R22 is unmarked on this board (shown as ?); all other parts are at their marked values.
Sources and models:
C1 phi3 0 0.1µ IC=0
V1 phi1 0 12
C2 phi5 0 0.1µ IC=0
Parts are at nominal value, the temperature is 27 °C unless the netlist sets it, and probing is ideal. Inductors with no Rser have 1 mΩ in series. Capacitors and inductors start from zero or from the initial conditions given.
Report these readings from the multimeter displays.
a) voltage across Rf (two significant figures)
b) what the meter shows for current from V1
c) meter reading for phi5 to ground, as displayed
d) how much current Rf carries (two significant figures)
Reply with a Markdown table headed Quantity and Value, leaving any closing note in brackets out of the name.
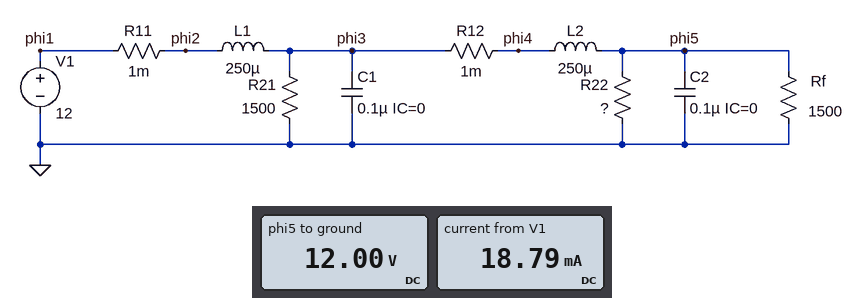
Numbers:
| Quantity | Value |
|---|---|
| voltage across Rf | 12 V |
| what the meter shows for current from V1 | 18.79 mA |
| meter reading for phi5 to ground, as displayed | 12.00 V |
| how much current Rf carries | 8.0 mA |
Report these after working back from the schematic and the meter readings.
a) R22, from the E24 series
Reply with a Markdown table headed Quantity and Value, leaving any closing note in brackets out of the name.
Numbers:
| Quantity | Value |
|---|---|
| R22, from the E24 series | 4.3 kΩ |
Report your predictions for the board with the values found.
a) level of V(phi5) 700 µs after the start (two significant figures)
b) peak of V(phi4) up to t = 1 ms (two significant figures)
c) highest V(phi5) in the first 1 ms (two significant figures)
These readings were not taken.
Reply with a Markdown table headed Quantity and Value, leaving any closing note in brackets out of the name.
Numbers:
| Quantity | Value |
|---|---|
| level of V(phi5) 700 µs after the start | 12 V |
| peak of V(phi4) up to t = 1 ms | 22 V |
| highest V(phi5) in the first 1 ms | 25 V |
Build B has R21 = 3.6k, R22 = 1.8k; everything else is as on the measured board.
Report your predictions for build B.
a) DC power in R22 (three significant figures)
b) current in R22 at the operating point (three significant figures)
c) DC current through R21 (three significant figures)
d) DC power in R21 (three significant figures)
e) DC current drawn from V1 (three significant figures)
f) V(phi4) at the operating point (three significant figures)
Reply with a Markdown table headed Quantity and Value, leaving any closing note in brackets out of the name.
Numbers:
| Quantity | Value |
|---|---|
| DC power in R22 | 80.0 mW |
| current in R22 at the operating point | 6.67 mA |
| DC current through R21 | 3.33 mA |
| DC power in R21 | 40.0 mW |
| DC current drawn from V1 | 18.0 mA |
| V(phi4) at the operating point | 12.0 V |
